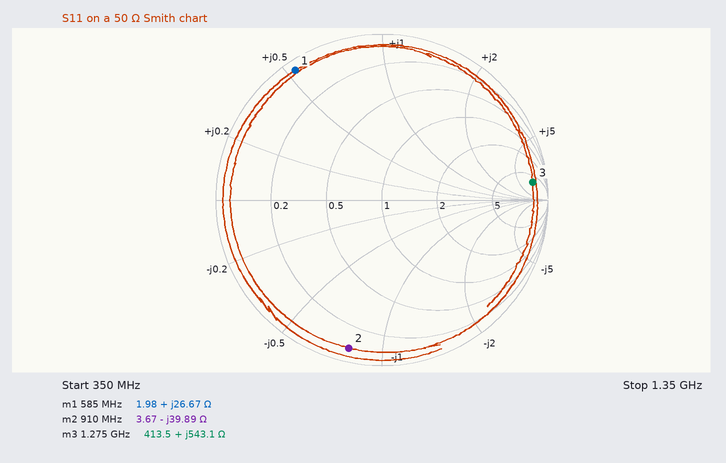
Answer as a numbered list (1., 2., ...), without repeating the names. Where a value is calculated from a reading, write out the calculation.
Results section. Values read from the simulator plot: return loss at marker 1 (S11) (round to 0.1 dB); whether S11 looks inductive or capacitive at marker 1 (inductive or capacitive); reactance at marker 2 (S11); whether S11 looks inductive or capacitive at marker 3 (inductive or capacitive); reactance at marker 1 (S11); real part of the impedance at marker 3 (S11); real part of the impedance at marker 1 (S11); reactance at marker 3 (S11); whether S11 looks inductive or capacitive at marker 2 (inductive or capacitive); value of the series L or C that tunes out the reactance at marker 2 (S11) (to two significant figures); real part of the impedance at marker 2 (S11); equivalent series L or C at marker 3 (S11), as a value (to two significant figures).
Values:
1. 0.5 dB
2. inductive
3. -39.89 Ω
4. inductive
5. +26.67 Ω
6. 413.5 Ω
7. 1.98 Ω
8. +543.1 Ω
9. capacitive
10. L = 39.89 Ω/(2π × 910 MHz) ≈ 7.0 nH
11. 3.67 Ω
12. L = 543.1 Ω/(2π × 1.275 GHz) ≈ 68 nH
